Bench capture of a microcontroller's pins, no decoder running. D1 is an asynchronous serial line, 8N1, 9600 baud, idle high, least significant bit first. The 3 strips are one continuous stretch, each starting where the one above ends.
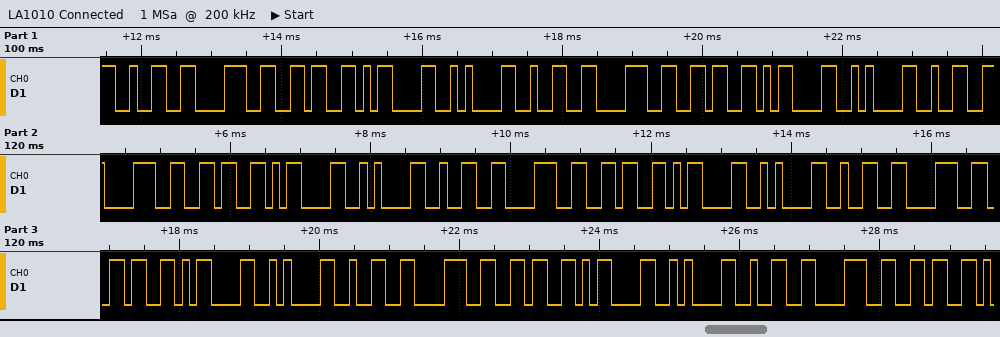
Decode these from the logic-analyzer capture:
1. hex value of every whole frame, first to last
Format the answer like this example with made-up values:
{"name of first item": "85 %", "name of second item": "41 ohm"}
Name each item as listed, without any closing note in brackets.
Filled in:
{"hex value of every whole frame, first to last": "0x32 0x38 0x36 0x0D 0x0A 0x32 0x38 0x36 0x0D 0x0A 0x32 0x38 0x36 0x0D 0x0A 0x32 0x38 0x36 0x0D 0x0A 0x32 0x38 0x36 0x0D 0x0A 0x32 0x38 0x36 0x0D 0x0A 0x32 0x38 0x36"}
